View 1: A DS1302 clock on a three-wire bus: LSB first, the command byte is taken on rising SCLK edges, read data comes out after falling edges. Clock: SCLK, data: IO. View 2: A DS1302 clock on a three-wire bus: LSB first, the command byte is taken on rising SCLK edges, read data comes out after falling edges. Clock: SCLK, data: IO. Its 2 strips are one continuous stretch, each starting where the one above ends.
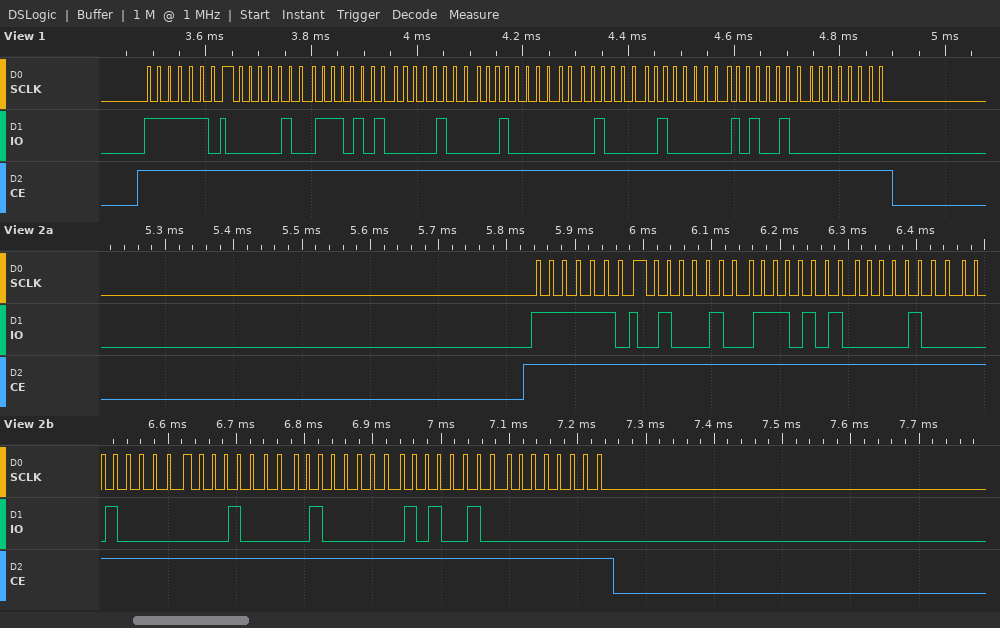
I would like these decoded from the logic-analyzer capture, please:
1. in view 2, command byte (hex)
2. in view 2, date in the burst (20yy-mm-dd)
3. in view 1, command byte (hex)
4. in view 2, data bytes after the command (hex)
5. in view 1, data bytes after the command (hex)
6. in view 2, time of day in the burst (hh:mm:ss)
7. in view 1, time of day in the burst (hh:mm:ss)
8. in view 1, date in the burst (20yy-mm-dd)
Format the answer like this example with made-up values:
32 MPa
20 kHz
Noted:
0xBF
2025-08-04
0xBF
22 57 10 04 08 02 25 00
20 57 10 04 08 02 25 00
10:57:22
10:57:20
2025-08-04
